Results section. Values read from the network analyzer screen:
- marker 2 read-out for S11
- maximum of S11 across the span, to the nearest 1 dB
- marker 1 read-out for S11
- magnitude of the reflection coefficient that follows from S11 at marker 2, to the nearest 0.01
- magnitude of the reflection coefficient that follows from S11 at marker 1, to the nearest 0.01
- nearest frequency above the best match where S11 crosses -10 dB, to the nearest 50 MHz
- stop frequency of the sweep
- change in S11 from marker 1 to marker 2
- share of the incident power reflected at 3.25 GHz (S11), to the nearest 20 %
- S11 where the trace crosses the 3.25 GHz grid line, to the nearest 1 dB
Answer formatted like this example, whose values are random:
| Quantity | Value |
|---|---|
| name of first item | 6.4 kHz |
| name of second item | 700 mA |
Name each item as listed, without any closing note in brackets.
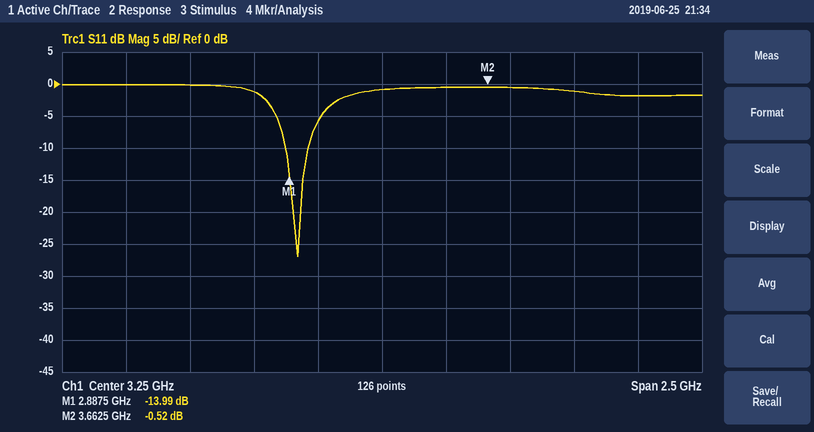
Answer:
| Quantity | Value |
|---|---|
| marker 2 read-out for S11 | -0.52 dB |
| maximum of S11 across the span, to the nearest 1 dB | 0 dB |
| marker 1 read-out for S11 | -13.99 dB |
| magnitude of the reflection coefficient that follows from S11 at marker 2, to the nearest 0.01 | 0.94 |
| magnitude of the reflection coefficient that follows from S11 at marker 1, to the nearest 0.01 | 0.20 |
| nearest frequency above the best match where S11 crosses -10 dB, to the nearest 50 MHz | 2.95 GHz |
| stop frequency of the sweep | 4.5 GHz |
| change in S11 from marker 1 to marker 2 | 13.47 dB |
| share of the incident power reflected at 3.25 GHz (S11), to the nearest 20 % | 80 % |
| S11 where the trace crosses the 3.25 GHz grid line, to the nearest 1 dB | -1 dB |
